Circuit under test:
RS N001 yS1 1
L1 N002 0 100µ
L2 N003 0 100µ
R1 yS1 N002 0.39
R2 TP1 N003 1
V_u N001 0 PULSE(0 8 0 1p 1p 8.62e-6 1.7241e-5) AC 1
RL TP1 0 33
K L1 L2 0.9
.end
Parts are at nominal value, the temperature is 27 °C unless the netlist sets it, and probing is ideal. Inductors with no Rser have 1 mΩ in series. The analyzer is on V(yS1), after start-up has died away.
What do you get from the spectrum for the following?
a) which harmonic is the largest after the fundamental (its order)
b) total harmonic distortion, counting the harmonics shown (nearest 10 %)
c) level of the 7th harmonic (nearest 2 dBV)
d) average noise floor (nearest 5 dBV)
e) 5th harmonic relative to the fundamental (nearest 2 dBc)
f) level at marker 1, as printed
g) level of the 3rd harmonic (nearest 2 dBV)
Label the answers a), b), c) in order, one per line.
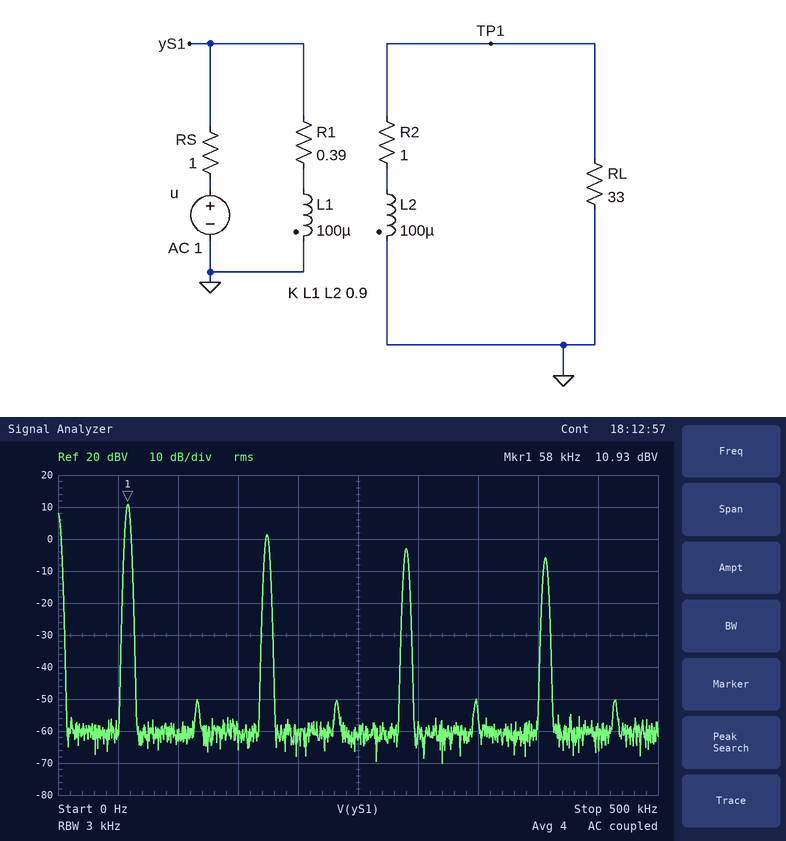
a) 3
b) 40 %
c) -6 dBV
d) -60 dBV
e) -14 dBc
f) 10.93 dBV
g) 2 dBV
